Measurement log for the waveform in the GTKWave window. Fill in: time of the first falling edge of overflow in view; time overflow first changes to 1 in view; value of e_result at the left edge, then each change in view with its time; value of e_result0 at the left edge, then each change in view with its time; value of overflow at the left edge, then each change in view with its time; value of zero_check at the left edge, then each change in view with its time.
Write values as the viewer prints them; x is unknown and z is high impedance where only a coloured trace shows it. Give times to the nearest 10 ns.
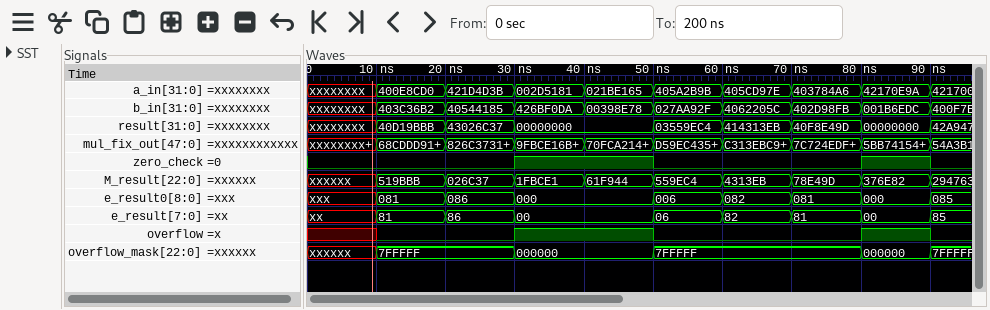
50 ns
30 ns
xx, 81 at 10 ns, 86 at 20 ns, 00 at 30 ns, 06 at 50 ns, 82 at 60 ns, 81 at 70 ns, 00 at 80 ns, 85 at 90 ns
xxx, 081 at 10 ns, 086 at 20 ns, 000 at 30 ns, 006 at 50 ns, 082 at 60 ns, 081 at 70 ns, 000 at 80 ns, 085 at 90 ns
x, 0 at 10 ns, 1 at 30 ns, 0 at 50 ns, 1 at 80 ns, 0 at 90 ns
0, 1 at 30 ns, 0 at 50 ns, 1 at 80 ns, 0 at 90 ns
